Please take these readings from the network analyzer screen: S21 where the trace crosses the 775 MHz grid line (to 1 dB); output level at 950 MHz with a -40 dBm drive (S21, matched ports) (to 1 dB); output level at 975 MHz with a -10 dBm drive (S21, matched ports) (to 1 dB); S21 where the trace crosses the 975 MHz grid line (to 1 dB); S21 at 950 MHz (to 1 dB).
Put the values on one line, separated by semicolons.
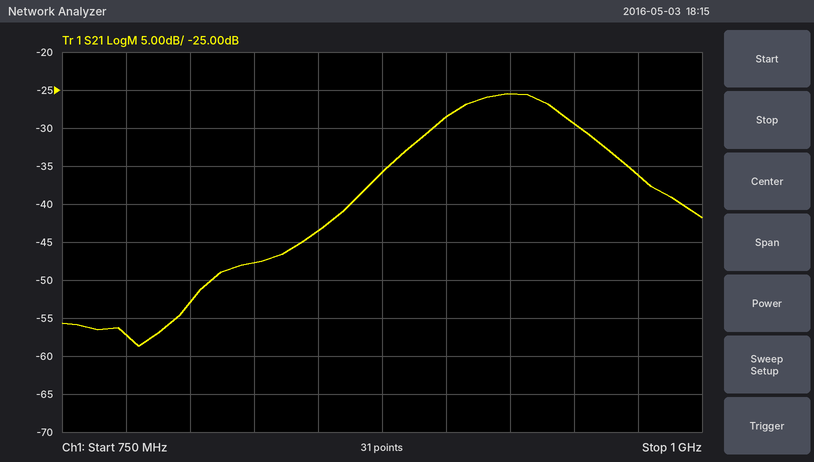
-57 dB; -69 dBm; -46 dBm; -36 dB; -29 dB
